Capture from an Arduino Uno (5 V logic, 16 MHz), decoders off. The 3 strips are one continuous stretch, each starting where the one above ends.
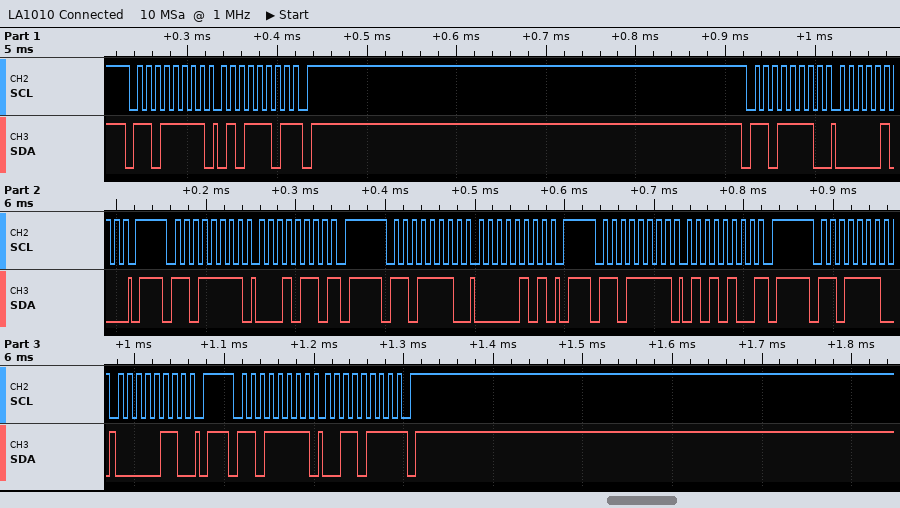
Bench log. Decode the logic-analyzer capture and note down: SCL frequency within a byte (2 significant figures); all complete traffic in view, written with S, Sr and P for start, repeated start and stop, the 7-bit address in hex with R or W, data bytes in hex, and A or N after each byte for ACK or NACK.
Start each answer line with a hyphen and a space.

- 100 kHz
- S 6FR A 5D N P S 6FW A 04 A P S 6FR A 16 N P S 6FW A 05 A P S 6FR A 54 N P S 6FW A 06 A P S 6FR A 37 N P
